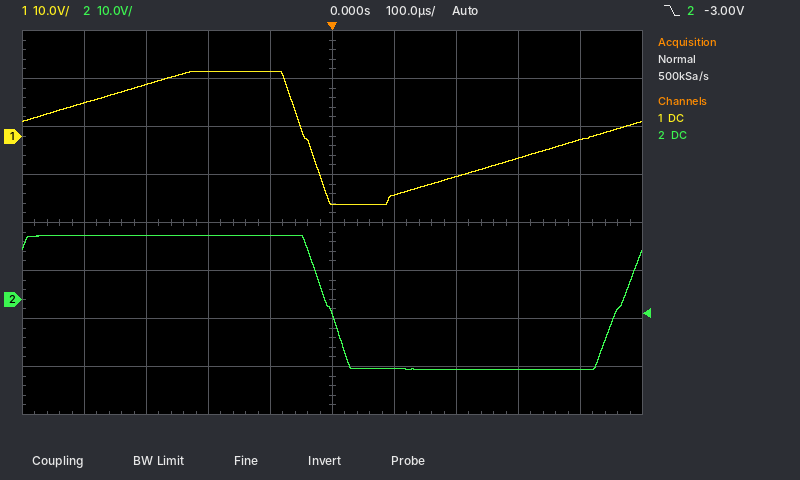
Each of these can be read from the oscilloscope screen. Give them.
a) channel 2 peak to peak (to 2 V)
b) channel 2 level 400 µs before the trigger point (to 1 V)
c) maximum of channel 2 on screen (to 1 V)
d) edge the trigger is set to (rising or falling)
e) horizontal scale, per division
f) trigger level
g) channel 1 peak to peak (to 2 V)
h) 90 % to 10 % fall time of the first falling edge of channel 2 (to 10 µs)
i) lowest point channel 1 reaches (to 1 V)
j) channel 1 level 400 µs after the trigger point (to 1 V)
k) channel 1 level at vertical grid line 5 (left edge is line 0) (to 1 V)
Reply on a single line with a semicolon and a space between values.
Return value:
28 V; 13 V; 13 V; falling; 100 µs; -3.00 V; 28 V; 60 µs; -14 V; -1 V; -14 V
